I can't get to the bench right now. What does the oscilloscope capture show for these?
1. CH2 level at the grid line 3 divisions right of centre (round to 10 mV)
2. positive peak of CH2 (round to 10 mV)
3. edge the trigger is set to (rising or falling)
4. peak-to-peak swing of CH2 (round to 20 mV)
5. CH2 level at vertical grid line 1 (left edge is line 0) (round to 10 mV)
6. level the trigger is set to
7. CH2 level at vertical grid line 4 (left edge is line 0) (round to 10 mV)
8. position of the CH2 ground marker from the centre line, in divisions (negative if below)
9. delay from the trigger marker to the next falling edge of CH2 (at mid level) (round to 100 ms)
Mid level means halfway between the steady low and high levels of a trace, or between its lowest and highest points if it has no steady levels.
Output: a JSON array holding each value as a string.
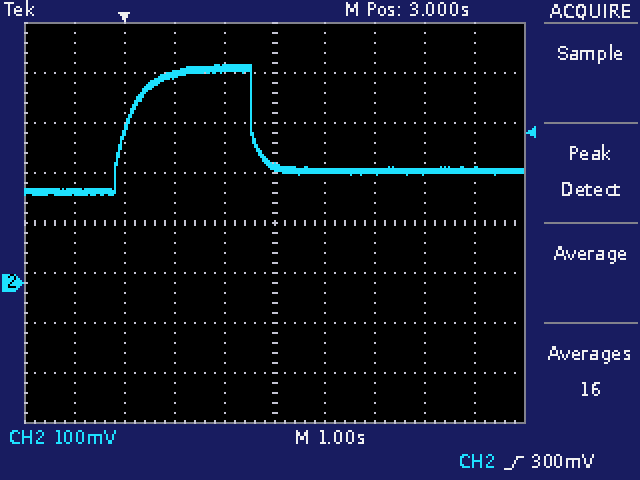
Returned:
["220 mV", "440 mV", "rising", "260 mV", "180 mV", "300 mV", "430 mV", "-1.2 div", "2.6 s"]
